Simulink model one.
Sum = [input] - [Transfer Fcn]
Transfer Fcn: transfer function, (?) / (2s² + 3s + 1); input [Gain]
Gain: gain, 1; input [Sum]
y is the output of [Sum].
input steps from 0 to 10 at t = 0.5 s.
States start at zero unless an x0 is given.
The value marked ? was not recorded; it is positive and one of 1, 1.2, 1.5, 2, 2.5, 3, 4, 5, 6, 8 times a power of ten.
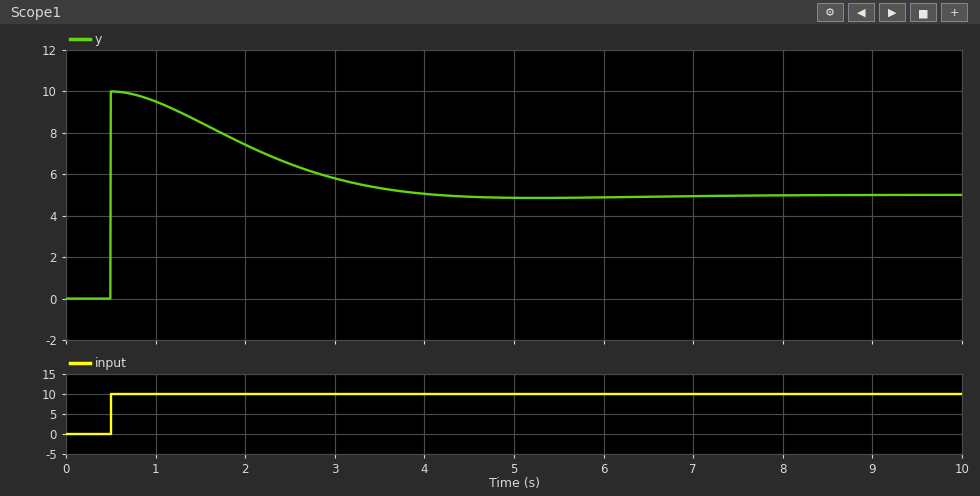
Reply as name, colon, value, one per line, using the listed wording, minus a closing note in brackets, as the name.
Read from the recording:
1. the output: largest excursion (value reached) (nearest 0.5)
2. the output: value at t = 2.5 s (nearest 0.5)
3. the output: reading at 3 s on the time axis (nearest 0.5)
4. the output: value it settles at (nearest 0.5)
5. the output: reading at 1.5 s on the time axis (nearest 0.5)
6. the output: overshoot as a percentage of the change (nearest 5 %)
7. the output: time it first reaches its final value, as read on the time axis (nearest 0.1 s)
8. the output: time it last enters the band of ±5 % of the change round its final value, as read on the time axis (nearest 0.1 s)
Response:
the output: largest excursion (value reached): 10.0
the output: value at t = 2.5 s: 6.5
the output: reading at 3 s on the time axis: 6.0
the output: value it settles at: 5.0
the output: reading at 1.5 s on the time axis: 8.5
the output: overshoot as a percentage of the change: 100 %
the output: time it first reaches its final value, as read on the time axis: 0.5 s
the output: time it last enters the band of ±5 % of the change round its final value, as read on the time axis: 3.6 s
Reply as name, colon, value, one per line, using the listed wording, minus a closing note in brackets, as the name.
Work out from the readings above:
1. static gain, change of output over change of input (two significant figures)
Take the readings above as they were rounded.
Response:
static gain, change of output over change of input: 0.50
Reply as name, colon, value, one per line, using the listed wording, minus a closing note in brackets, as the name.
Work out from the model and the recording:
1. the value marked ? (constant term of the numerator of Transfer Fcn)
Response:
the value marked ?: 1
